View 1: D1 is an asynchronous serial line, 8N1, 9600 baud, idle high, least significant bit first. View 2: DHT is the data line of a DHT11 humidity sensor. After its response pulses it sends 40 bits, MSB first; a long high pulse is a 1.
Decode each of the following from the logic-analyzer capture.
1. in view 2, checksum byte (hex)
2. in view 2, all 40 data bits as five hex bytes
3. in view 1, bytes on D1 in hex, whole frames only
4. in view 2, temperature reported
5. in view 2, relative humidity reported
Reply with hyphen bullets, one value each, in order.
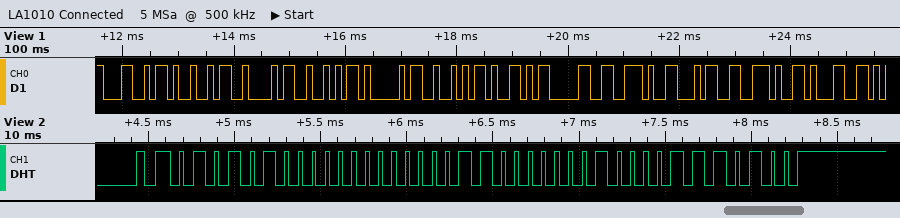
- 0x74
- 54 00 18 08 74
- 4C 49 42 52 41 52 59 30 2E 34 2E 31
- 24.8 °C
- 84 %
